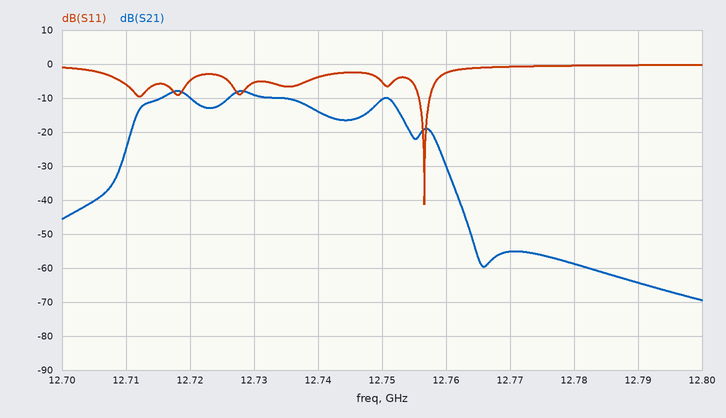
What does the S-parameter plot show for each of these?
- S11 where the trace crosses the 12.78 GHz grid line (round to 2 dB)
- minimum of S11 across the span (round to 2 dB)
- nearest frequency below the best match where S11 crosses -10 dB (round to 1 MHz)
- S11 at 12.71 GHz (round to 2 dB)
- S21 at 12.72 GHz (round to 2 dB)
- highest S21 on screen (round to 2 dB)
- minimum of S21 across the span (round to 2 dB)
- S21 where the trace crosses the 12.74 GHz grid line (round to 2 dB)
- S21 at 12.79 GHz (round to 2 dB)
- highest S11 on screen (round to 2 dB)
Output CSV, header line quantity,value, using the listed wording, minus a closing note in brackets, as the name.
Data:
quantity,value
S11 where the trace crosses the 12.78 GHz grid line,0 dB
minimum of S11 across the span,-42 dB
nearest frequency below the best match where S11 crosses -10 dB,12.756 GHz
S11 at 12.71 GHz,-6 dB
S21 at 12.72 GHz,-10 dB
highest S21 on screen,-8 dB
minimum of S21 across the span,-70 dB
S21 where the trace crosses the 12.74 GHz grid line,-14 dB
S21 at 12.79 GHz,-64 dB
highest S11 on screen,0 dB
